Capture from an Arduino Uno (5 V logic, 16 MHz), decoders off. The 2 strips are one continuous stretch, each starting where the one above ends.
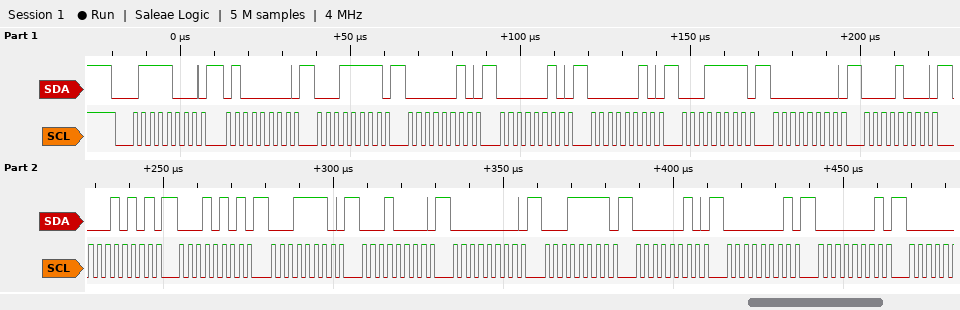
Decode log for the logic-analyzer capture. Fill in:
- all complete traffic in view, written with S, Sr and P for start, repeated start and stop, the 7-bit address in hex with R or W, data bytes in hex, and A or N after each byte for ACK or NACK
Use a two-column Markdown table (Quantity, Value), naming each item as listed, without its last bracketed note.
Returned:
| Quantity | Value |
|---|---|
| all complete traffic in view, written with S, Sr and P for start, repeated start and stop, the 7-bit address in hex with R or W, data bytes in hex, and A or N after each byte for ACK or NACK | S 3CW A 40 A 1F A 02 A 02 A 02 A 1F A 00 A 08 A 15 A 15 A 1E A 10 A 00 A 1F A 02 A 01 A 01 A |
